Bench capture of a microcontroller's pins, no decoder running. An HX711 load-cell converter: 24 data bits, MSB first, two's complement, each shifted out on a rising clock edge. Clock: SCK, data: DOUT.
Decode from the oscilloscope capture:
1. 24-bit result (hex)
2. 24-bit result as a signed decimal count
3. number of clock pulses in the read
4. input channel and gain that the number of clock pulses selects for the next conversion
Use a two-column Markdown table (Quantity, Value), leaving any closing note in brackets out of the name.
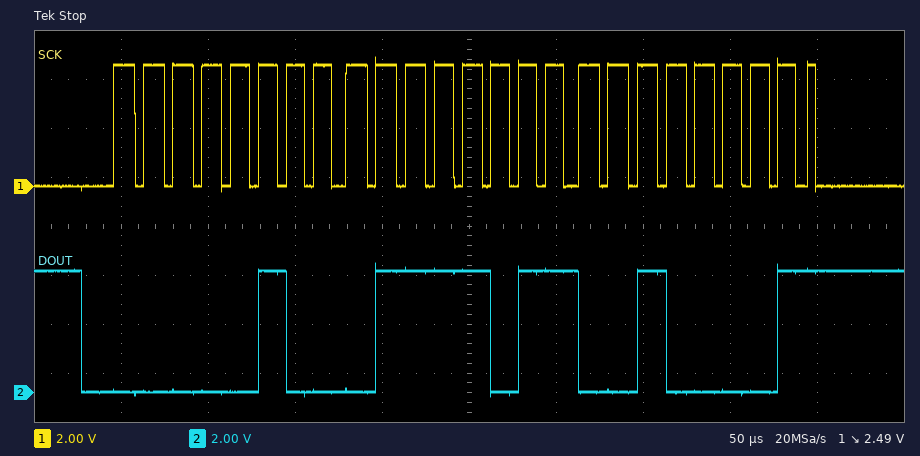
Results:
| Quantity | Value |
|---|---|
| 24-bit result | 0x047B21 |
| 24-bit result as a signed decimal count | 293665 |
| number of clock pulses in the read | 25 |
| input channel and gain that the number of clock pulses selects for the next conversion | channel A, gain 128 |
